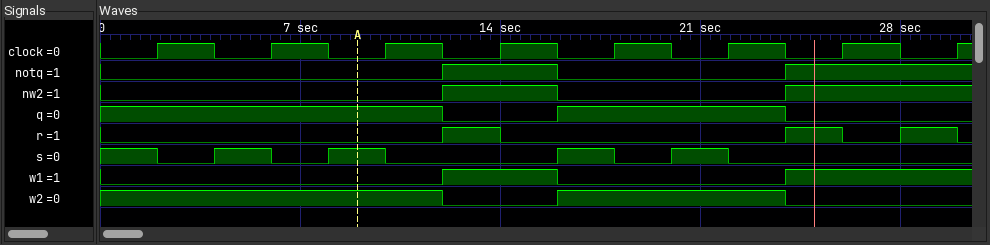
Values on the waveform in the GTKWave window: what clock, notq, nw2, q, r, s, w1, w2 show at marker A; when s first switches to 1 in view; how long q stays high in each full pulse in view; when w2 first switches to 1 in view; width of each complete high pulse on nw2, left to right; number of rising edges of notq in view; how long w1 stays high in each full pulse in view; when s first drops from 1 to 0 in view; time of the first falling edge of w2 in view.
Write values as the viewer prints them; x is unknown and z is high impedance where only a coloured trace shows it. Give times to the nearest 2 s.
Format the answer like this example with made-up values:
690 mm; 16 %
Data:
clock=0, notq=0, nw2=0, q=1, r=0, s=1, w1=0, w2=1; 4 s; 8 s; 16 s; 4 s; 2; 4 s; 2 s; 12 s
